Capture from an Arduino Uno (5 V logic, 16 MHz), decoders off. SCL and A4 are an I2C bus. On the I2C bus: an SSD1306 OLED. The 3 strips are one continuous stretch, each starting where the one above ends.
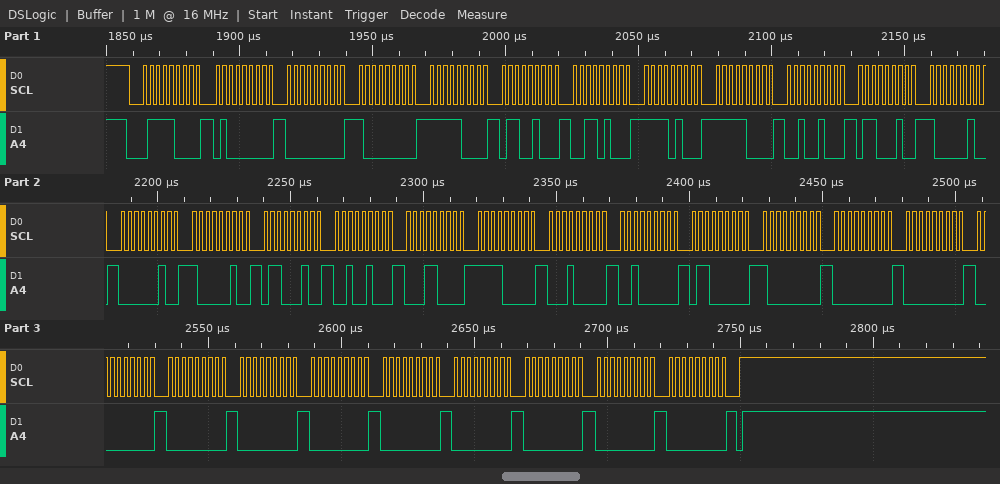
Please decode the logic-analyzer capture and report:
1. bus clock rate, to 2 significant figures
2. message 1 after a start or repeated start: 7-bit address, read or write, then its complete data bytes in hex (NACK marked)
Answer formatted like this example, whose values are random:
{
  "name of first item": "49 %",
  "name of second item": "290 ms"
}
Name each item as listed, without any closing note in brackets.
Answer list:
{
  "bus clock rate, to 2 significant figures": "400 kHz",
  "message 1 after a start or repeated start: 7-bit address, read or write, then its complete data bytes in hex": "0x3C write: 40 00 80 F8 64 34 F4 F8 24 62 82 02 82 62 24 18 F0 10 20 60 80 00 00 00 00 00 00 00 00 00 00 00"
}
